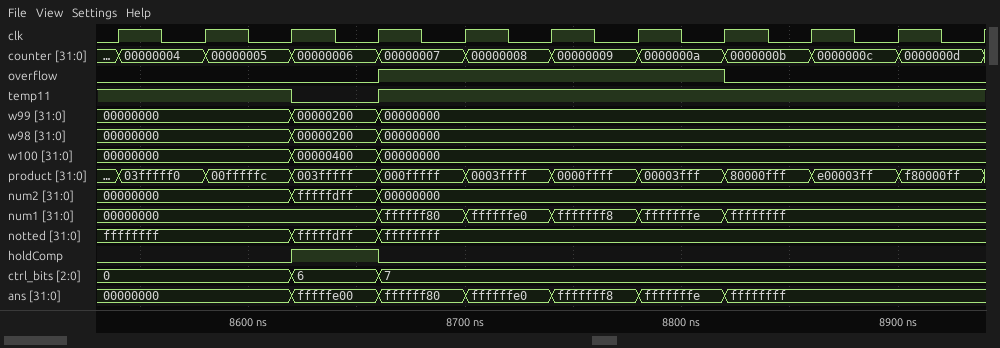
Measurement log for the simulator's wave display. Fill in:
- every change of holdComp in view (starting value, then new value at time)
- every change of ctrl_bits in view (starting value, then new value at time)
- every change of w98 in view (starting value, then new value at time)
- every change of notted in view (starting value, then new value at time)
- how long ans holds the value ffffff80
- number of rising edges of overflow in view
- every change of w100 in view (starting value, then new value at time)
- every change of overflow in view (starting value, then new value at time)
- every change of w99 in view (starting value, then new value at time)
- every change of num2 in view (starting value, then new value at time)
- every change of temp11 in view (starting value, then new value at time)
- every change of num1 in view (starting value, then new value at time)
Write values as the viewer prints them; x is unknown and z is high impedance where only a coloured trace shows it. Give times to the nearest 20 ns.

0, 1 at 8620 ns, 0 at 8660 ns
0, 6 at 8620 ns, 7 at 8660 ns
00000000, 00000200 at 8620 ns, 00000000 at 8660 ns
ffffffff, fffffdff at 8620 ns, ffffffff at 8660 ns
40 ns
1
00000000, 00000400 at 8620 ns, 00000000 at 8660 ns
0, 1 at 8660 ns, 0 at 8820 ns
00000000, 00000200 at 8620 ns, 00000000 at 8660 ns
00000000, fffffdff at 8620 ns, 00000000 at 8660 ns
1, 0 at 8620 ns, 1 at 8660 ns
00000000, ffffff80 at 8660 ns, ffffffe0 at 8700 ns, fffffff8 at 8740 ns, fffffffe at 8780 ns, ffffffff at 8820 ns
